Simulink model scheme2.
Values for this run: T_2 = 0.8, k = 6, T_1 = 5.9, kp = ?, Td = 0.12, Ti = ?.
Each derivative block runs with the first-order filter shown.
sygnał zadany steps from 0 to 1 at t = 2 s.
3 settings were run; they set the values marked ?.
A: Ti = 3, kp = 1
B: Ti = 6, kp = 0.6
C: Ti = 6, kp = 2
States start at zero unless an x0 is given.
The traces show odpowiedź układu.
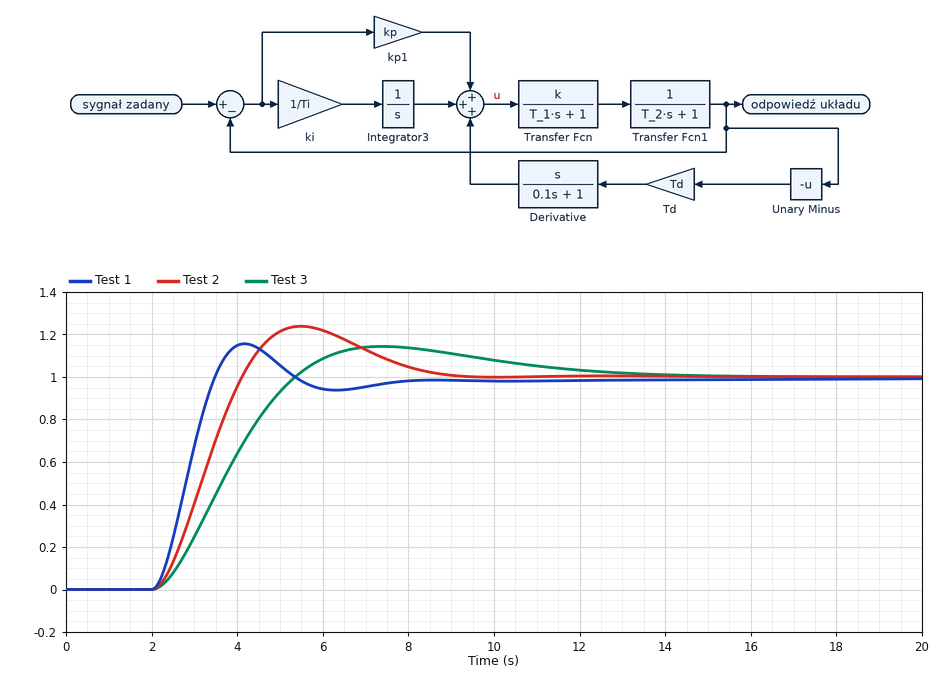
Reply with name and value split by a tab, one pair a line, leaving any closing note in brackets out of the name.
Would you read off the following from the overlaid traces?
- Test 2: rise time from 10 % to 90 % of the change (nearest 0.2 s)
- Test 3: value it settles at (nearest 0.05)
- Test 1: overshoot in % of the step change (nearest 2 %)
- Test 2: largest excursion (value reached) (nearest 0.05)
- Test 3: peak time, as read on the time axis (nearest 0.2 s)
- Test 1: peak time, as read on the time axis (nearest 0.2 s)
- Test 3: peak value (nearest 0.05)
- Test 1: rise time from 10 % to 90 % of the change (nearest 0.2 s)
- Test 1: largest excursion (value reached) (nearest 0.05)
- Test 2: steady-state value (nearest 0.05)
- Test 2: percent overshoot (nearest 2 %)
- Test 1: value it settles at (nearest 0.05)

Test 2: rise time from 10 % to 90 % of the change	1.4 s
Test 3: value it settles at	1.00
Test 1: overshoot in % of the step change	16 %
Test 2: largest excursion (value reached)	1.25
Test 3: peak time, as read on the time axis	7.4 s
Test 1: peak time, as read on the time axis	4.2 s
Test 3: peak value	1.15
Test 1: rise time from 10 % to 90 % of the change	1.0 s
Test 1: largest excursion (value reached)	1.15
Test 2: steady-state value	1.00
Test 2: percent overshoot	24 %
Test 1: value it settles at	1.00
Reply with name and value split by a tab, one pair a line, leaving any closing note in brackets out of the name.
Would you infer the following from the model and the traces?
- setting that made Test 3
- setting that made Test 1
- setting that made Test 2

setting that made Test 3	B
setting that made Test 1	C
setting that made Test 2	A
